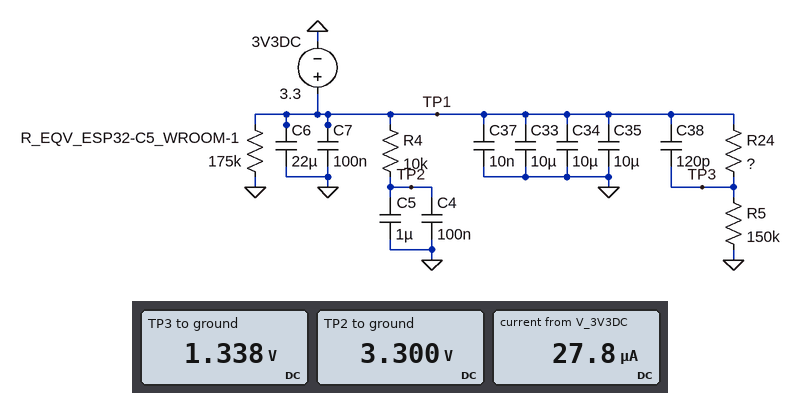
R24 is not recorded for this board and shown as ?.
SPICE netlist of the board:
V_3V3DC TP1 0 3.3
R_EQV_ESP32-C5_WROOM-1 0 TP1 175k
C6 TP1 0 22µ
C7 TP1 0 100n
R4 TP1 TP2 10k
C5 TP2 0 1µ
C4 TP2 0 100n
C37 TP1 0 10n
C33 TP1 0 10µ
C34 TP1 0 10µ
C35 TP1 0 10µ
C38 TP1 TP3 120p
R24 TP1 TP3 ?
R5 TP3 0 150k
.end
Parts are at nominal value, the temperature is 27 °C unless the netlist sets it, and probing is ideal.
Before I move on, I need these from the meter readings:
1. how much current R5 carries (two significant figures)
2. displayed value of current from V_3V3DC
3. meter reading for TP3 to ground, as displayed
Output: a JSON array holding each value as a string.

["8.9 µA", "27.8 µA", "1.338 V"]
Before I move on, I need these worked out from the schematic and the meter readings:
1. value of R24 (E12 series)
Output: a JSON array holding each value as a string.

["220 kΩ"]
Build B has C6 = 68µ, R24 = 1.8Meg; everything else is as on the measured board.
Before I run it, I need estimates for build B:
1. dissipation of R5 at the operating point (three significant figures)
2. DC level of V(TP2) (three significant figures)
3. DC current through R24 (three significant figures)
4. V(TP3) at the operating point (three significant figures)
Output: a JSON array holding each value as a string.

["430 nW", "3.30 V", "1.69 µA", "254 mV"]
